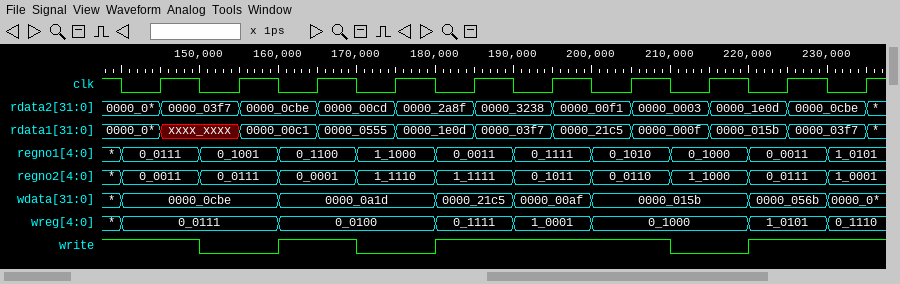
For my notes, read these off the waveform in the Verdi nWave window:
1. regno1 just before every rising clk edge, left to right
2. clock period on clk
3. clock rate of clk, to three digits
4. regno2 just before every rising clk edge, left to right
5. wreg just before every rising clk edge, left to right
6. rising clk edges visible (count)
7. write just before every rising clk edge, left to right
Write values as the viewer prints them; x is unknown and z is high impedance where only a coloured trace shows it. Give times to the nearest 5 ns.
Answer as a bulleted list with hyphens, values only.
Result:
- 0_0111, 0_1001, 0_1100, 1_1000, 0_0011, 0_1111, 0_1010, 0_1000, 0_0011, 1_0101
- 10 ns
- 100 MHz
- 0_0011, 0_0111, 0_0001, 1_1110, 1_1111, 0_1011, 0_0110, 1_1000, 0_0111, 1_0001
- 0_0111, 0_0111, 0_0100, 0_0100, 0_1111, 1_0001, 0_1000, 0_1000, 1_0101, 0_1110
- 10
- 1 0 1 0 1 1 1 0 1 1
